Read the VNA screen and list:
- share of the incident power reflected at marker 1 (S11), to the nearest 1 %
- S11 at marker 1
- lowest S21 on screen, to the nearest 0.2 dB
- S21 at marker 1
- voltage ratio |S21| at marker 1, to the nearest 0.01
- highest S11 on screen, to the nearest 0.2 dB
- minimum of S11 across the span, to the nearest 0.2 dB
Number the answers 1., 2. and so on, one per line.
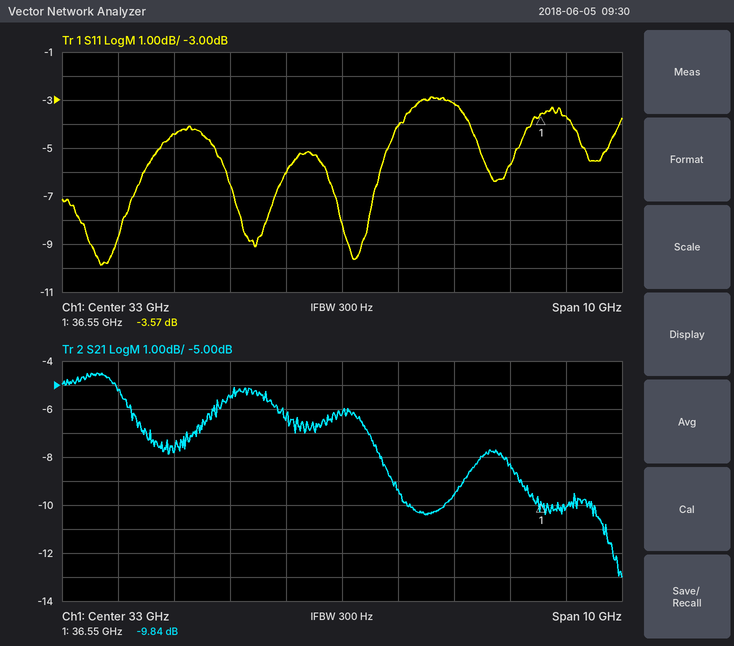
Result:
1. 44 %
2. -3.57 dB
3. -13.0 dB
4. -9.84 dB
5. 0.32
6. -2.8 dB
7. -9.8 dB
